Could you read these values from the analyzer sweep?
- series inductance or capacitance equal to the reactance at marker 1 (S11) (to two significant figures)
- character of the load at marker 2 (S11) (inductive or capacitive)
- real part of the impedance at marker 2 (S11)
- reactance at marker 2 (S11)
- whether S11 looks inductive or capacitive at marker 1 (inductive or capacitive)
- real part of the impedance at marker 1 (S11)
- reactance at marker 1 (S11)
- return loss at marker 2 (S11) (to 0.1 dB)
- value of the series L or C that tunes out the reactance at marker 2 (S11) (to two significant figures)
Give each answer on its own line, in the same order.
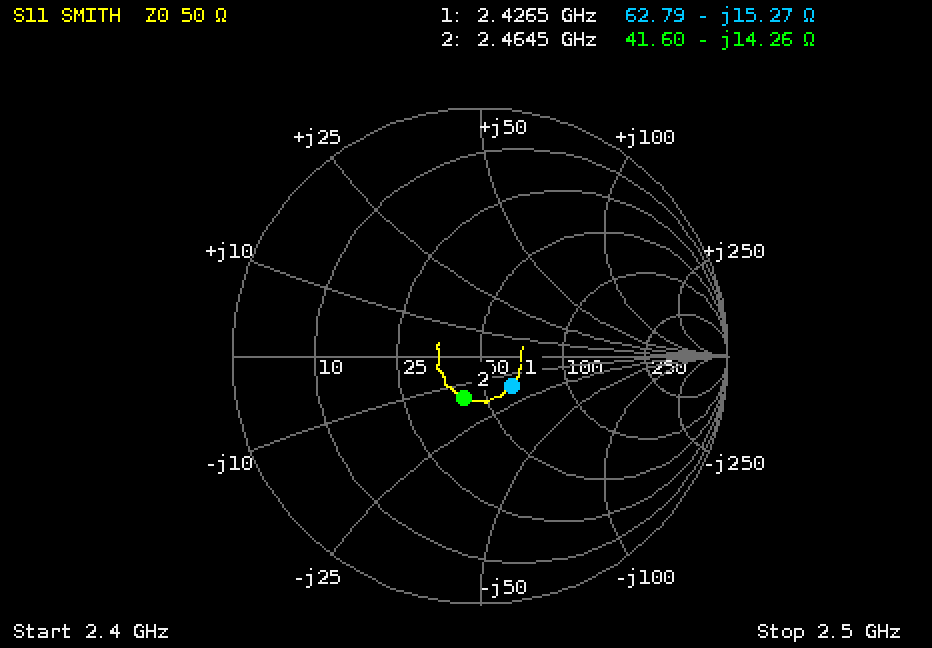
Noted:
4.3 pF
capacitive
41.60 Ω
-14.26 Ω
capacitive
62.79 Ω
-15.27 Ω
15.0 dB
920 pH
